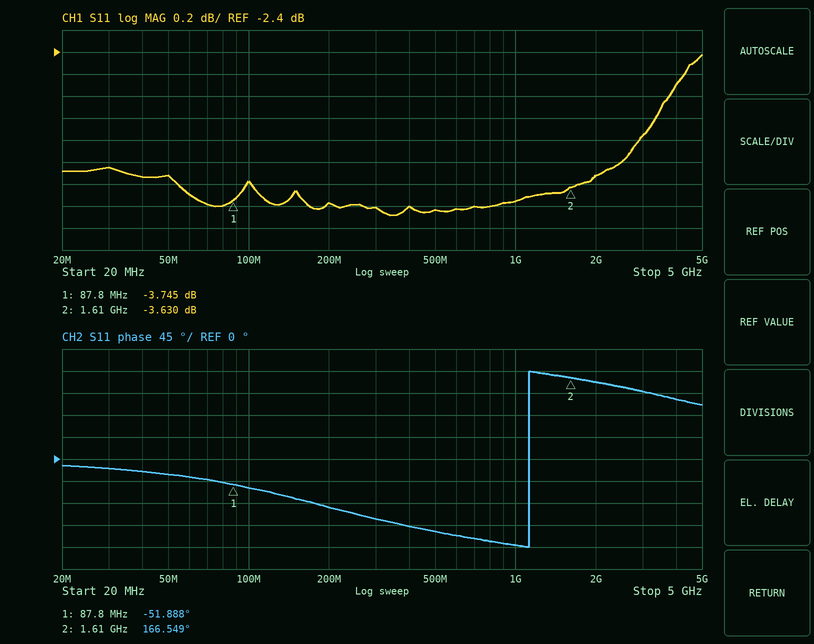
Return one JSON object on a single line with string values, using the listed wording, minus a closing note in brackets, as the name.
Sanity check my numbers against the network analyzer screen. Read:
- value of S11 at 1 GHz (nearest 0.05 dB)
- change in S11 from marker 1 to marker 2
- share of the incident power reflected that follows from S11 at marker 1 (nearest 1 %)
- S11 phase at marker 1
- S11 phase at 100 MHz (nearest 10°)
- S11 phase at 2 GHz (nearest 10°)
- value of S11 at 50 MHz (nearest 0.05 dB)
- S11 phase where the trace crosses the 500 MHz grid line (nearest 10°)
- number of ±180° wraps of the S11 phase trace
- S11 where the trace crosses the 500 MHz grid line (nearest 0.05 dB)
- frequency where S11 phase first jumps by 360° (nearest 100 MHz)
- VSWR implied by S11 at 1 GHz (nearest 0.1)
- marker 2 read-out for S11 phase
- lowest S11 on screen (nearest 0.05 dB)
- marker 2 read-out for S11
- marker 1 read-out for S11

{"value of S11 at 1 GHz": "-3.75 dB", "change in S11 from marker 1 to marker 2": "0.115 dB", "share of the incident power reflected that follows from S11 at marker 1": "42 %", "S11 phase at marker 1": "-51.888°", "S11 phase at 100 MHz": "-60°", "S11 phase at 2 GHz": "160°", "value of S11 at 50 MHz": "-3.50 dB", "S11 phase where the trace crosses the 500 MHz grid line": "-150°", "number of ±180° wraps of the S11 phase trace": "1", "S11 where the trace crosses the 500 MHz grid line": "-3.85 dB", "frequency where S11 phase first jumps by 360°": "1.1 GHz", "VSWR implied by S11 at 1 GHz": "4.7", "marker 2 read-out for S11 phase": "166.549°", "lowest S11 on screen": "-3.90 dB", "marker 2 read-out for S11": "-3.630 dB", "marker 1 read-out for S11": "-3.745 dB"}
